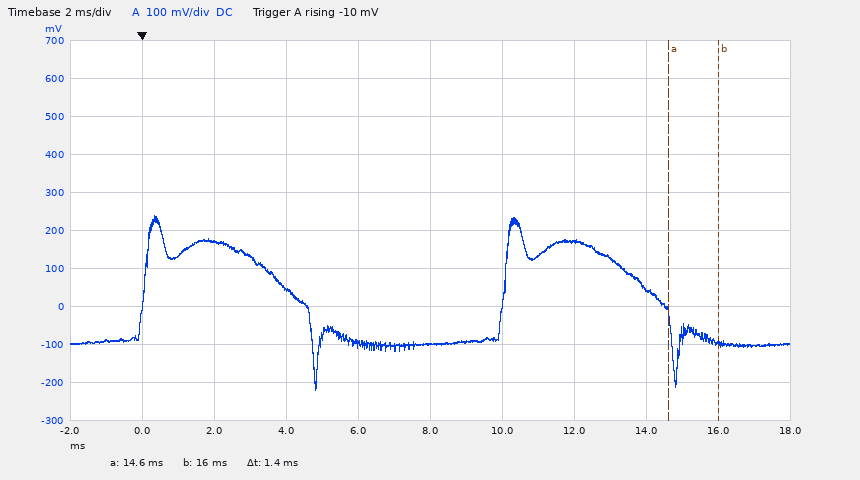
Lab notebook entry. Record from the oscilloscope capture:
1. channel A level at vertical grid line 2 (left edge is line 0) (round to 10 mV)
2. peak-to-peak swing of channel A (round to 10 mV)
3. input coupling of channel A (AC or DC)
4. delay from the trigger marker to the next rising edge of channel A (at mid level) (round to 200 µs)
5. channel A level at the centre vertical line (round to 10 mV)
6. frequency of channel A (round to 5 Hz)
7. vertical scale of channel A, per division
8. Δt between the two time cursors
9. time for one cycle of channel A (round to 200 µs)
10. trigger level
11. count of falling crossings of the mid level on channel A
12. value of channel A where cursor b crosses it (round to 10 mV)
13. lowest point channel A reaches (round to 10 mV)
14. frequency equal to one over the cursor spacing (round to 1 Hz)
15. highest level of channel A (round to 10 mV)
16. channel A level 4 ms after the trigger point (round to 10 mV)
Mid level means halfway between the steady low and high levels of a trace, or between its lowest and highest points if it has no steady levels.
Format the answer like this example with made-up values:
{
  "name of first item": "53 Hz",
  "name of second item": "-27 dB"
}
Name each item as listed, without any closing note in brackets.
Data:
{
  "channel A level at vertical grid line 2 (left edge is line 0)": "170 mV",
  "peak-to-peak swing of channel A": "460 mV",
  "input coupling of channel A": "DC",
  "delay from the trigger marker to the next rising edge of channel A (at mid level)": "10.0 ms",
  "channel A level at the centre vertical line": "-100 mV",
  "frequency of channel A": "100 Hz",
  "vertical scale of channel A, per division": "100 mV",
  "Δt between the two time cursors": "1.4 ms",
  "time for one cycle of channel A": "10.0 ms",
  "trigger level": "-10 mV",
  "count of falling crossings of the mid level on channel A": "2",
  "value of channel A where cursor b crosses it": "-100 mV",
  "lowest point channel A reaches": "-220 mV",
  "frequency equal to one over the cursor spacing": "714 Hz",
  "highest level of channel A": "240 mV",
  "channel A level 4 ms after the trigger point": "50 mV"
}
